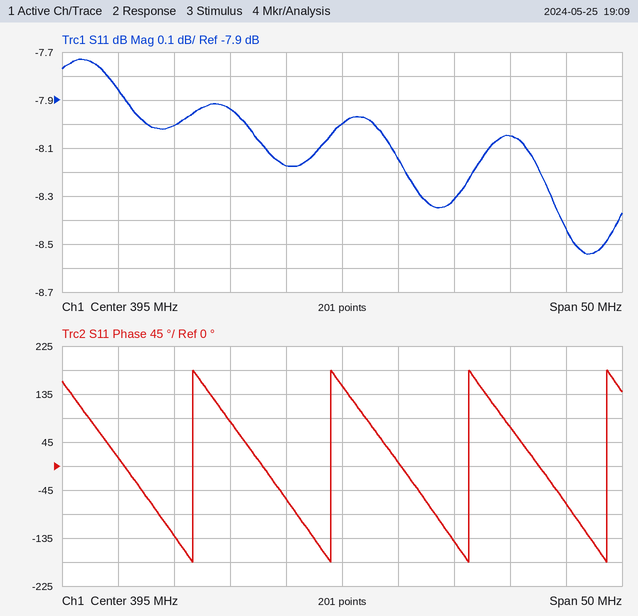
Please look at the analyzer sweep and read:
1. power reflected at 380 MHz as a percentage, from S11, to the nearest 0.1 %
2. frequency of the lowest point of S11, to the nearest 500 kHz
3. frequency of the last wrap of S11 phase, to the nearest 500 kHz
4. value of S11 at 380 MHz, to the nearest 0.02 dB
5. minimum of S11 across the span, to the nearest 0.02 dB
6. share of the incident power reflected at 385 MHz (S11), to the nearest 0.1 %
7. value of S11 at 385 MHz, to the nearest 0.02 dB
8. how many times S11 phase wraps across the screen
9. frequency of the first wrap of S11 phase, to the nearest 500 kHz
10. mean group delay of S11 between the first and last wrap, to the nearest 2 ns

15.8 %
417.0 MHz
418.5 MHz
-8.00 dB
-8.54 dB
16.1 %
-7.94 dB
4
381.5 MHz
82 ns
